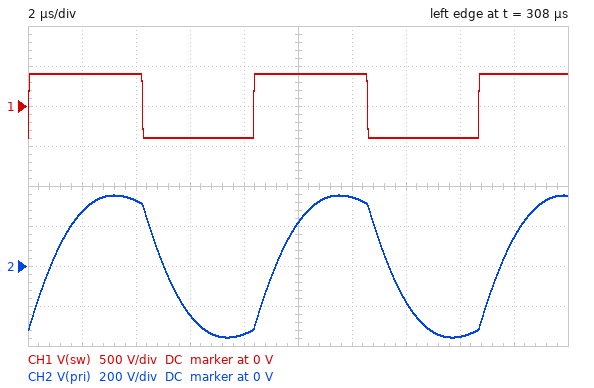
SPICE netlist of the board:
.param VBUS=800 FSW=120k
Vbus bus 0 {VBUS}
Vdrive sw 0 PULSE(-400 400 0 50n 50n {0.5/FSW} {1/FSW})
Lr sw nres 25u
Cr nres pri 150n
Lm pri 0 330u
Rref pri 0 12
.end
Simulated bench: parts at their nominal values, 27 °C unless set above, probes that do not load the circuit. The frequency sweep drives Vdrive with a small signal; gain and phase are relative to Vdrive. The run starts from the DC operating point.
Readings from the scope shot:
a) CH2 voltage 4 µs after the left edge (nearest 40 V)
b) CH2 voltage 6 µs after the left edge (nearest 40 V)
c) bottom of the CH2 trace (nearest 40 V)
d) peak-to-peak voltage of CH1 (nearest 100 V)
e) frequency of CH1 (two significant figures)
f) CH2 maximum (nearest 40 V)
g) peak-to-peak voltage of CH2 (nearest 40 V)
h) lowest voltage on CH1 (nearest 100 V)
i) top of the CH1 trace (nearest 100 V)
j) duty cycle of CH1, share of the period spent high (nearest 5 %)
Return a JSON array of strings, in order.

["320 V", "-240 V", "-360 V", "800 V", "120 kHz", "360 V", "720 V", "-400 V", "400 V", "50 %"]
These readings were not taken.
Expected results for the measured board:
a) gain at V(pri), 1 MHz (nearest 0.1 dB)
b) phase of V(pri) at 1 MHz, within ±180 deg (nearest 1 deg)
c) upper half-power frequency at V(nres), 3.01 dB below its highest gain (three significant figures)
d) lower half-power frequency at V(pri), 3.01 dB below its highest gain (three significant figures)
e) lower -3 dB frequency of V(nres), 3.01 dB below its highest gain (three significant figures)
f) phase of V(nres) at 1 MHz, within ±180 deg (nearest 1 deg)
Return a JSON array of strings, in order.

["-22.3 dB", "-85 deg", "108 kHz", "50.1 kHz", "19.8 kHz", "-90 deg"]
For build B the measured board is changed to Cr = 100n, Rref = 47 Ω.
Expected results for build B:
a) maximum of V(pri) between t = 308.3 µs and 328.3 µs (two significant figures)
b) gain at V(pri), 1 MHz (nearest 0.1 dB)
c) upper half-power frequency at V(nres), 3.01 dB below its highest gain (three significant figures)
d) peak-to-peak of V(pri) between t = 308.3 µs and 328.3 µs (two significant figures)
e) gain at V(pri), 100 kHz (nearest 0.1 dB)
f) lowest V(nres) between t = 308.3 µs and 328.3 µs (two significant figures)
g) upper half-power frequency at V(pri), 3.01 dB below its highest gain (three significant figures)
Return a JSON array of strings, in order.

["440 V", "-10.8 dB", "264 kHz", "890 V", "0 dB", "-420 V", "263 kHz"]
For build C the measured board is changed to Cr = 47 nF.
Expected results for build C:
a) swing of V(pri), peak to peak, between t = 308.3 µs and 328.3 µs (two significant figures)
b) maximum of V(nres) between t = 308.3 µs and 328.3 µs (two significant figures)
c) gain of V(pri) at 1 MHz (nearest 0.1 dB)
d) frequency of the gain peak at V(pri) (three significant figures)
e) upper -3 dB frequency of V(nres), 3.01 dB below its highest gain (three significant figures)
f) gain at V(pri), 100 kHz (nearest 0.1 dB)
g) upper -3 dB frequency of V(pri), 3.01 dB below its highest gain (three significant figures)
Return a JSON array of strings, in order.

["900 V", "1.0 kV", "-22.2 dB", "145 kHz", "174 kHz", "-4.9 dB", "188 kHz"]
